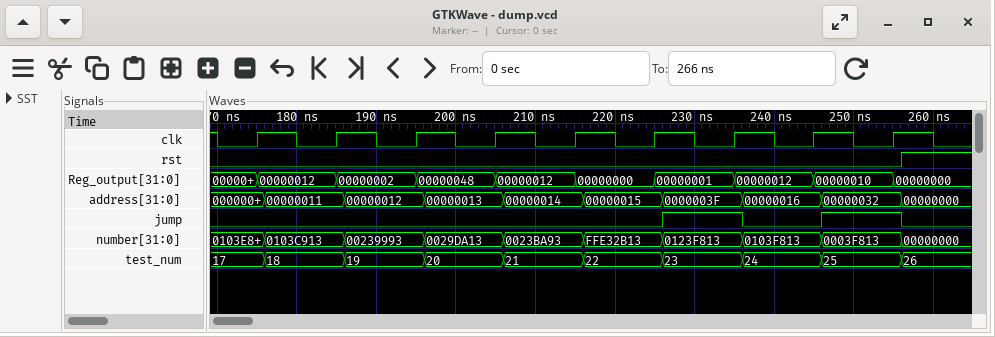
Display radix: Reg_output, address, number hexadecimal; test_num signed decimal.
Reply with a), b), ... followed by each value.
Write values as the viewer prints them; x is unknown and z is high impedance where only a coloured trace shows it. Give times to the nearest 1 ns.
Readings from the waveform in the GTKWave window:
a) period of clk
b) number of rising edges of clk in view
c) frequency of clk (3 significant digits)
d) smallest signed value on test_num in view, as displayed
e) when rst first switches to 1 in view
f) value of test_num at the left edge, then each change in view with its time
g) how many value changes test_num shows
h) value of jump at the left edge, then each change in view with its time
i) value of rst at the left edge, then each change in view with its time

a) 10 ns
b) 9
c) 100 MHz
d) 17
e) 256 ns
f) 17, 18 at 176 ns, 19 at 186 ns, 20 at 196 ns, 21 at 206 ns, 22 at 216 ns, 23 at 226 ns, 24 at 236 ns, 25 at 246 ns, 26 at 256 ns
g) 9
h) 0, 1 at 226 ns, 0 at 236 ns, 1 at 246 ns, 0 at 256 ns
i) 0, 1 at 256 ns
